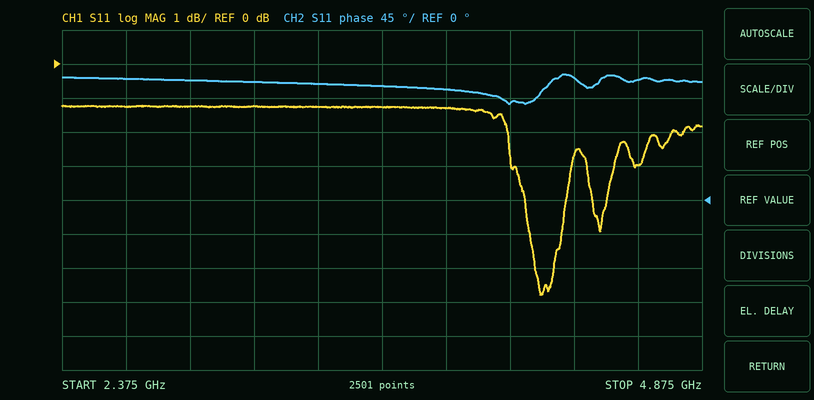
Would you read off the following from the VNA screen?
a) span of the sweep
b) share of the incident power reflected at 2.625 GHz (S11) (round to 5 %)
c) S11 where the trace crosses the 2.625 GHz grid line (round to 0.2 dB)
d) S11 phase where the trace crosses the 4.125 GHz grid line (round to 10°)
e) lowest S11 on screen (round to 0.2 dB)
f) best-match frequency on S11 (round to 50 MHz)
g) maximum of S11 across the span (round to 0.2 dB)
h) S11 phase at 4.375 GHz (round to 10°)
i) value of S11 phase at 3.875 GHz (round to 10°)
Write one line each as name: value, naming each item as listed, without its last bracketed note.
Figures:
span of the sweep: 2.5 GHz
share of the incident power reflected at 2.625 GHz (S11): 75 %
S11 where the trace crosses the 2.625 GHz grid line: -1.2 dB
S11 phase where the trace crosses the 4.125 GHz grid line: 130°
lowest S11 on screen: -6.8 dB
best-match frequency on S11: 4.25 GHz
maximum of S11 across the span: -1.2 dB
S11 phase at 4.375 GHz: 160°
value of S11 phase at 3.875 GHz: 150°
